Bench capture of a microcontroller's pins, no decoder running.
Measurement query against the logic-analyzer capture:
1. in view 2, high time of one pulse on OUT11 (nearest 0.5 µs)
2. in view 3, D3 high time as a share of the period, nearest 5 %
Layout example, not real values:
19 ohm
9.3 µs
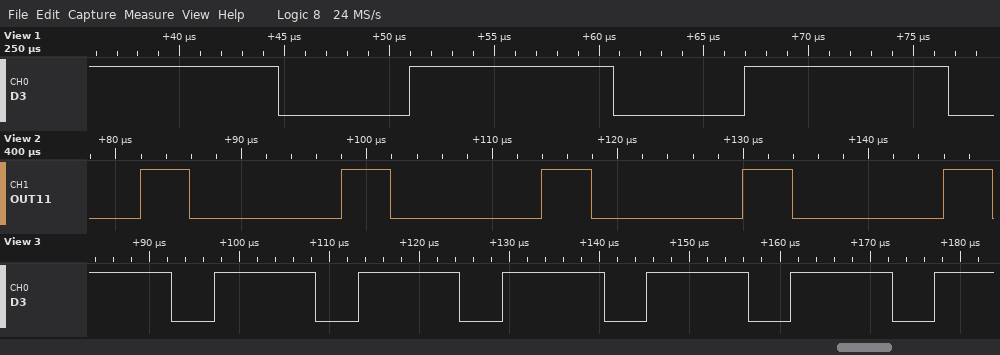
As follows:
4.0 µs
70 %
